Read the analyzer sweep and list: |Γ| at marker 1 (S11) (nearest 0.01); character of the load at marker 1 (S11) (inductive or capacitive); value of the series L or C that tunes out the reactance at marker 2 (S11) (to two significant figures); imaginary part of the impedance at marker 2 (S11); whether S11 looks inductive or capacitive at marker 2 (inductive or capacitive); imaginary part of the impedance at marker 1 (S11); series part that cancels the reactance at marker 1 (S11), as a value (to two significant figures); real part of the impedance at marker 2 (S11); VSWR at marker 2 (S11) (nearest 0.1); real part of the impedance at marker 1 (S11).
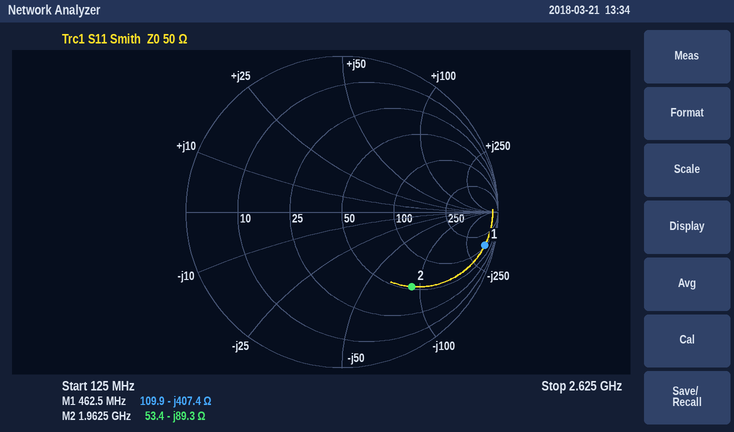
0.94
capacitive
7.2 nH
-89.3 Ω
capacitive
-407.4 Ω
140 nH
53.4 Ω
4.8
109.9 Ω
